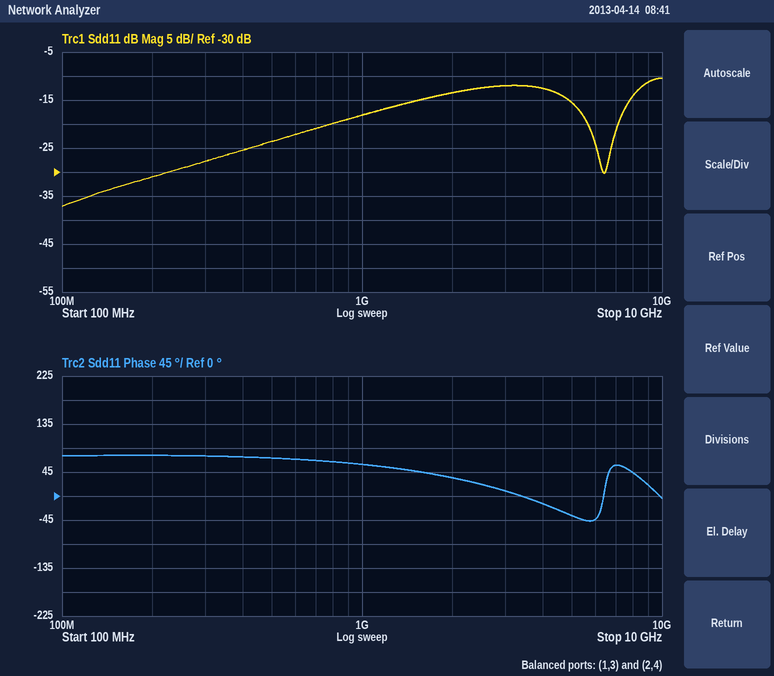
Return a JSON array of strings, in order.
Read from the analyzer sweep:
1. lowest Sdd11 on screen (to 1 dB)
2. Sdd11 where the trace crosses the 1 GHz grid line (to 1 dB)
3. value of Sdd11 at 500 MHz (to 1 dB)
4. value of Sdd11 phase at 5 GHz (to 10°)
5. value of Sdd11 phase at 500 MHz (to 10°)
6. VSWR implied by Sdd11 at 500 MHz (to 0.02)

["-37 dB", "-18 dB", "-24 dB", "-40°", "70°", "1.14"]
